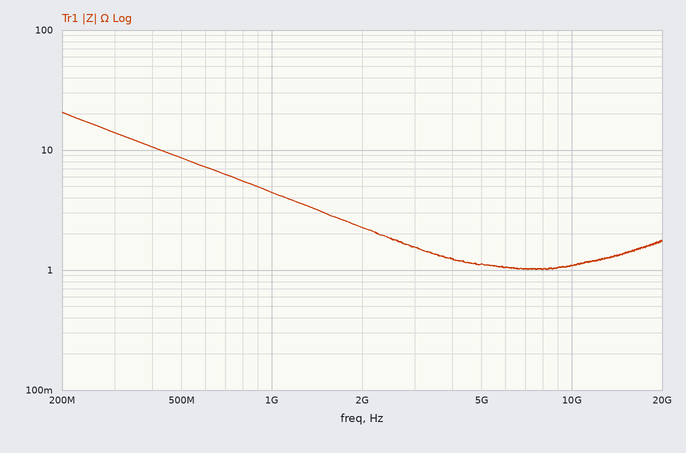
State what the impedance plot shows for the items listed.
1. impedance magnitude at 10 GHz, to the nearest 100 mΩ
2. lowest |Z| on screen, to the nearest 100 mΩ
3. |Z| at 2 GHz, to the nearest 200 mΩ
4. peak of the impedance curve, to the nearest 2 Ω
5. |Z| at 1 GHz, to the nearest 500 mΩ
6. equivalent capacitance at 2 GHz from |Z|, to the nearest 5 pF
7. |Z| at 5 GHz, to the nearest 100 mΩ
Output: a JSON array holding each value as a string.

["1.1 Ω", "1.0 Ω", "2.2 Ω", "20 Ω", "4.5 Ω", "35 pF", "1.1 Ω"]
